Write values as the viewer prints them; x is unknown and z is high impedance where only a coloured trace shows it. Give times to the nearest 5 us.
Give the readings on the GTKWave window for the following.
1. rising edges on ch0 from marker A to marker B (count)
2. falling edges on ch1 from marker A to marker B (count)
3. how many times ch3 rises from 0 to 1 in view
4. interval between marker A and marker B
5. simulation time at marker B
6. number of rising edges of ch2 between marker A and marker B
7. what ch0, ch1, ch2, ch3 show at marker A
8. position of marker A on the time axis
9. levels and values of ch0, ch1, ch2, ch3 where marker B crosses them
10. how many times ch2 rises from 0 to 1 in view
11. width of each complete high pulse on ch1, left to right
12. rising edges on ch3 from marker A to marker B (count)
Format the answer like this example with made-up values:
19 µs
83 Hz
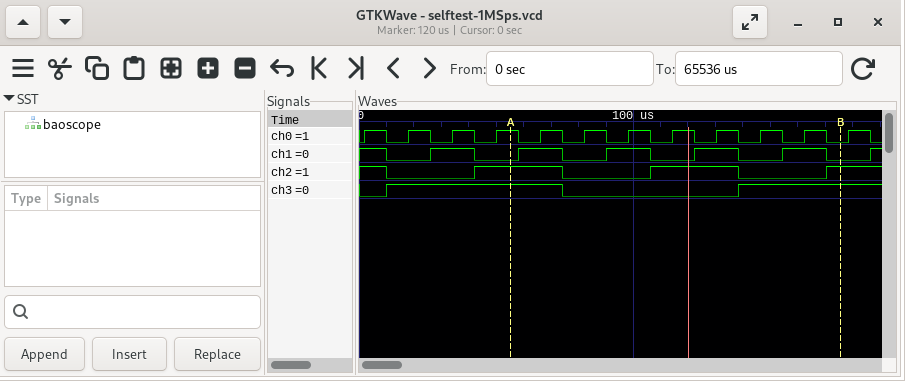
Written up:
7
4
2
120 us
175 us
2
ch0=1, ch1=0, ch2=1, ch3=1
55 us
ch0=0, ch1=0, ch2=1, ch3=1
3
15 us, 15 us, 15 us, 15 us, 15 us
1
